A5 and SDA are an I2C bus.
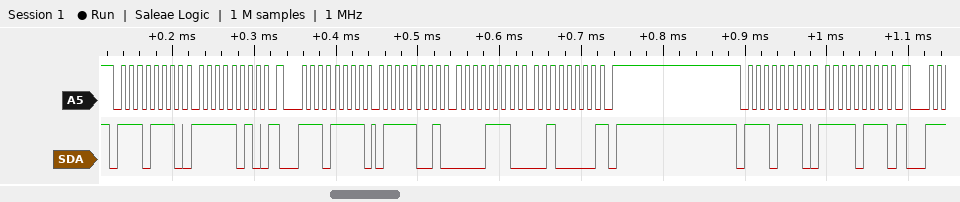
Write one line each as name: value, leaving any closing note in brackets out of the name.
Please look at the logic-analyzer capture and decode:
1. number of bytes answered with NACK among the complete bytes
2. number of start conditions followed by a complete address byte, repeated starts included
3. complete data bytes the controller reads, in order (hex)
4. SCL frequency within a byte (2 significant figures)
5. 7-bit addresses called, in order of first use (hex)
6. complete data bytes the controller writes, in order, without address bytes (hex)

number of bytes answered with NACK among the complete bytes: 1
number of start conditions followed by a complete address byte, repeated starts included: 3
complete data bytes the controller reads, in order: 79 0E 20
SCL frequency within a byte: 100 kHz
7-bit addresses called, in order of first use: 0x77
complete data bytes the controller writes, in order, without address bytes: FA F7
